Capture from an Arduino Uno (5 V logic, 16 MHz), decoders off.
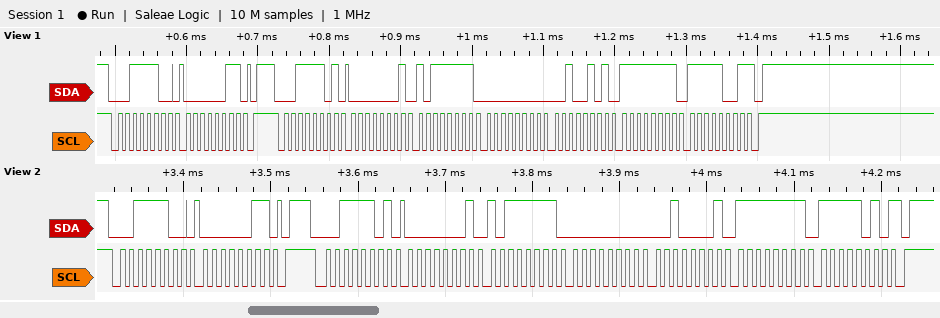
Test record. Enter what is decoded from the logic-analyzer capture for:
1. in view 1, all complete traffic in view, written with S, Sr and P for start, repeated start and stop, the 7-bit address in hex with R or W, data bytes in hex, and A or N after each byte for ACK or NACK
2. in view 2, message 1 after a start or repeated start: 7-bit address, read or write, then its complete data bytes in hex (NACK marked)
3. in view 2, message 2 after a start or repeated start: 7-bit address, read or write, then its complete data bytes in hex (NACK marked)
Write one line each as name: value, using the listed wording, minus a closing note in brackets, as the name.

in view 1, all complete traffic in view, written with S, Sr and P for start, repeated start and stop, the 7-bit address in hex with R or W, data bytes in hex, and A or N after each byte for ACK or NACK: S 1EW A 03 A P S 1ER A 01 A BF A 00 A 25 A FF A F9 N P
in view 2, message 1 after a start or repeated start: 7-bit address, read or write, then its complete data bytes in hex: 0x1E write: 03
in view 2, message 2 after a start or repeated start: 7-bit address, read or write, then its complete data bytes in hex: 0x1E read: 01 BF 00 21 FF FA NACK
